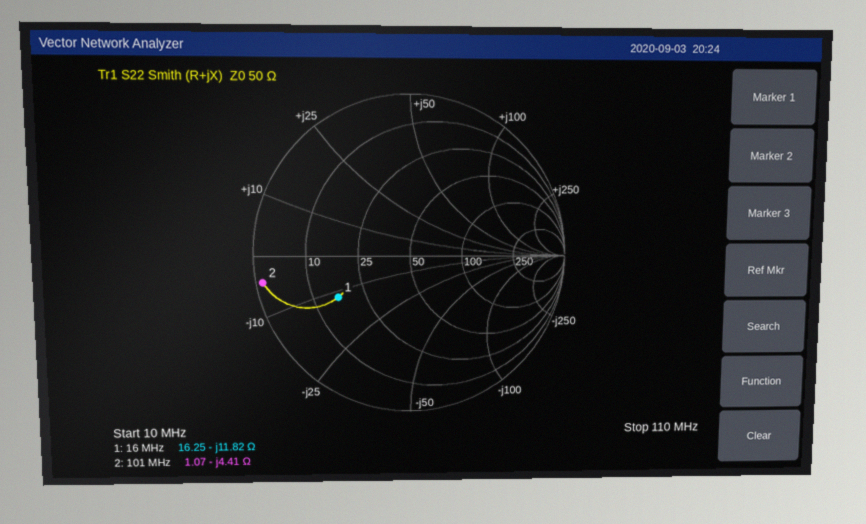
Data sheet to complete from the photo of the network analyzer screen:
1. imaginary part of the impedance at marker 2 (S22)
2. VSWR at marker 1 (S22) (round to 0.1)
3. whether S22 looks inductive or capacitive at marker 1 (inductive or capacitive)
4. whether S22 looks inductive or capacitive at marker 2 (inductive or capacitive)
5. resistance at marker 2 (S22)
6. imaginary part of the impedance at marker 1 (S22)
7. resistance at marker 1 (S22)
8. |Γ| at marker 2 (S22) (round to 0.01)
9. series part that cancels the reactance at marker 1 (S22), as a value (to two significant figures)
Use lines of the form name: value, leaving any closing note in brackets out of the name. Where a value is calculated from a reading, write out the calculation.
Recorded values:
imaginary part of the impedance at marker 2: -4.41 Ω
VSWR at marker 1 (S22): 3.3
whether S22 looks inductive or capacitive at marker 1: capacitive
whether S22 looks inductive or capacitive at marker 2: capacitive
resistance at marker 2: 1.07 Ω
imaginary part of the impedance at marker 1: -11.82 Ω
resistance at marker 1: 16.25 Ω
|Γ| at marker 2 (S22): 0.96
series part that cancels the reactance at marker 1 (S22), as a value: L = 11.82 Ω/(2π × 16 MHz) ≈ 118 nH, so 120 nH to two significant figures
